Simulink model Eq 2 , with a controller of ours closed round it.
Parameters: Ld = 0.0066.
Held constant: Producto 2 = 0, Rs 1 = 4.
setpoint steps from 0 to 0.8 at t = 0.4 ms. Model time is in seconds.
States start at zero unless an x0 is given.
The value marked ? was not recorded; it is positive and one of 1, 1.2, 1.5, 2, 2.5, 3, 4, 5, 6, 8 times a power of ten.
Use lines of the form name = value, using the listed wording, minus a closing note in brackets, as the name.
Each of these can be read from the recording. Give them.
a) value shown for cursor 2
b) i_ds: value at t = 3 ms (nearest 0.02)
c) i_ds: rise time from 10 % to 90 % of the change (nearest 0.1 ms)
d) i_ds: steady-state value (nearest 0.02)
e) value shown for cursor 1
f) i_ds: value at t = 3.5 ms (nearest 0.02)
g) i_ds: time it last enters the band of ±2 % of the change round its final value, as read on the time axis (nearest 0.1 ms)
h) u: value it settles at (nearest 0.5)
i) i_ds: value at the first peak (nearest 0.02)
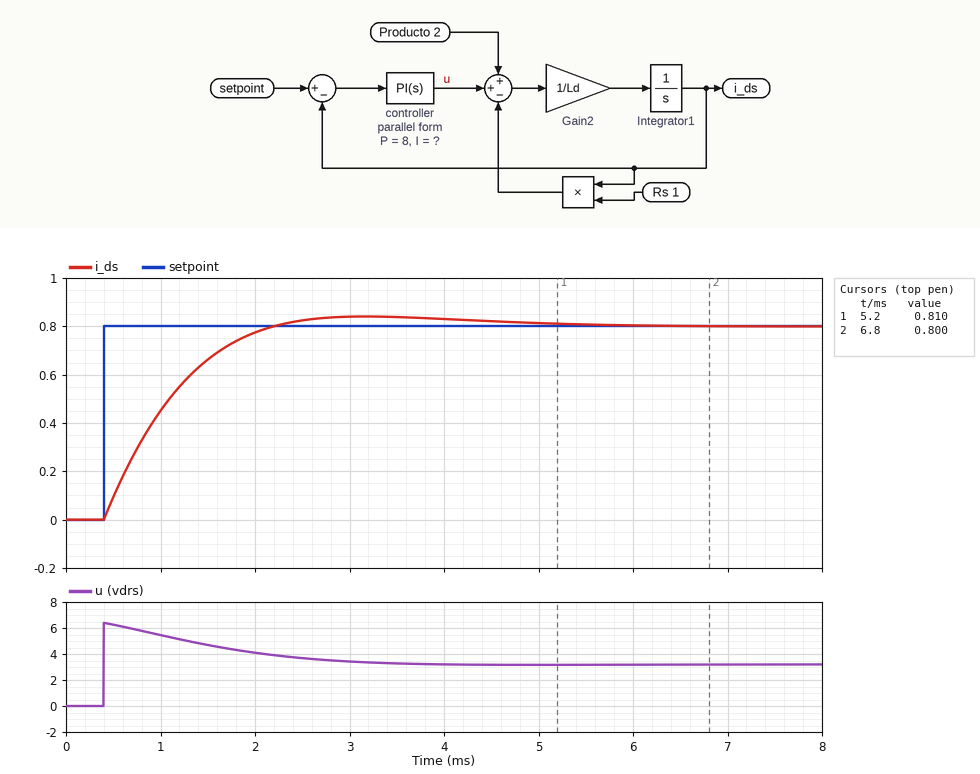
value shown for cursor 2 = 0.800
i_ds: value at t = 3 ms = 0.84
i_ds: rise time from 10 % to 90 % of the change = 1.2 ms
i_ds: steady-state value = 0.80
value shown for cursor 1 = 0.810
i_ds: value at t = 3.5 ms = 0.84
i_ds: time it last enters the band of ±2 % of the change round its final value, as read on the time axis = 4.8 ms
u: value it settles at = 3.0
i_ds: value at the first peak = 0.84
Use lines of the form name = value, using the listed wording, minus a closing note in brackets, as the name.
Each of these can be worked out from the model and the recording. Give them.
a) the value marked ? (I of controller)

the value marked ? = 8000
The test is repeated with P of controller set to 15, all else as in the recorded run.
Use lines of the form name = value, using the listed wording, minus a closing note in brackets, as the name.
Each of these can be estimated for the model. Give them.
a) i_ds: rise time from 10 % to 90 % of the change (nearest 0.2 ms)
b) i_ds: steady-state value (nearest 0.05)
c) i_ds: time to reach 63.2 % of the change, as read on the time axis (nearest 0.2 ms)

i_ds: rise time from 10 % to 90 % of the change = 1.0 ms
i_ds: steady-state value = 0.80
i_ds: time to reach 63.2 % of the change, as read on the time axis = 0.8 ms
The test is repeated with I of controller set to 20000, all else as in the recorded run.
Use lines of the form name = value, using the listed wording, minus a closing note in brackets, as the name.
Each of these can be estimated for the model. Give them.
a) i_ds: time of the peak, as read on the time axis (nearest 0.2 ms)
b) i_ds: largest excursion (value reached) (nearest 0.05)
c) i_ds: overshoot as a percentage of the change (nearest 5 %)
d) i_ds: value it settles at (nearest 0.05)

i_ds: time of the peak, as read on the time axis = 2.0 ms
i_ds: largest excursion (value reached) = 0.95
i_ds: overshoot as a percentage of the change = 20 %
i_ds: value it settles at = 0.80
